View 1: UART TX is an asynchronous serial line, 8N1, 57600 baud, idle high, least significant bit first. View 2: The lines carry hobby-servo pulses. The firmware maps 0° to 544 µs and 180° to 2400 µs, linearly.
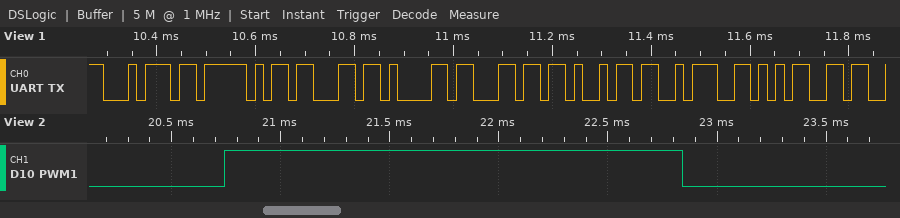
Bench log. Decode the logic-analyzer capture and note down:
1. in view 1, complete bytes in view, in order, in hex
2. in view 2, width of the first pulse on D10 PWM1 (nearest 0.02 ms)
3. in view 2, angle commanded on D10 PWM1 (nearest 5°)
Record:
0x74 0x5F 0x63 0x61 0x6C 0x69 0x3A 0x35
2.10 ms
150°
